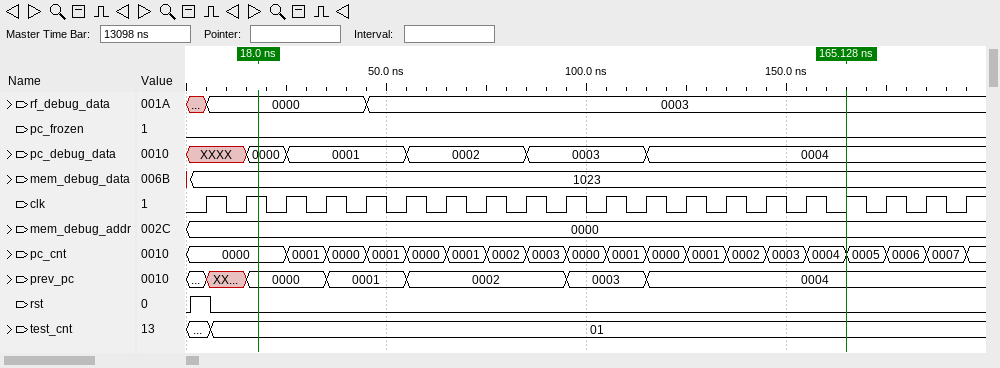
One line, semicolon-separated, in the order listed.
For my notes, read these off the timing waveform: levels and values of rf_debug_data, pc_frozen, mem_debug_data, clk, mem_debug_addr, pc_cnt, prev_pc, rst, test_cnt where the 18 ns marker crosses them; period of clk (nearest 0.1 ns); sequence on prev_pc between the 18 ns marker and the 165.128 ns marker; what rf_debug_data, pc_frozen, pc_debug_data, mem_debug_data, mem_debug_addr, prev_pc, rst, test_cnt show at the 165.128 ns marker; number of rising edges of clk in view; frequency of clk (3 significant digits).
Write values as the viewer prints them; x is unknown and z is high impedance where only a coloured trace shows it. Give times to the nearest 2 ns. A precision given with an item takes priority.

rf_debug_data=0000, pc_frozen=0, mem_debug_data=1023, clk=1, mem_debug_addr=0000, pc_cnt=0000, prev_pc=0000, rst=0, test_cnt=01; 10 ns; 0000, 0001, 0002, 0003, 0004; rf_debug_data=0003, pc_frozen=0, pc_debug_data=0004, mem_debug_data=1023, mem_debug_addr=0000, prev_pc=0004, rst=0, test_cnt=01; 20; 100 MHz
